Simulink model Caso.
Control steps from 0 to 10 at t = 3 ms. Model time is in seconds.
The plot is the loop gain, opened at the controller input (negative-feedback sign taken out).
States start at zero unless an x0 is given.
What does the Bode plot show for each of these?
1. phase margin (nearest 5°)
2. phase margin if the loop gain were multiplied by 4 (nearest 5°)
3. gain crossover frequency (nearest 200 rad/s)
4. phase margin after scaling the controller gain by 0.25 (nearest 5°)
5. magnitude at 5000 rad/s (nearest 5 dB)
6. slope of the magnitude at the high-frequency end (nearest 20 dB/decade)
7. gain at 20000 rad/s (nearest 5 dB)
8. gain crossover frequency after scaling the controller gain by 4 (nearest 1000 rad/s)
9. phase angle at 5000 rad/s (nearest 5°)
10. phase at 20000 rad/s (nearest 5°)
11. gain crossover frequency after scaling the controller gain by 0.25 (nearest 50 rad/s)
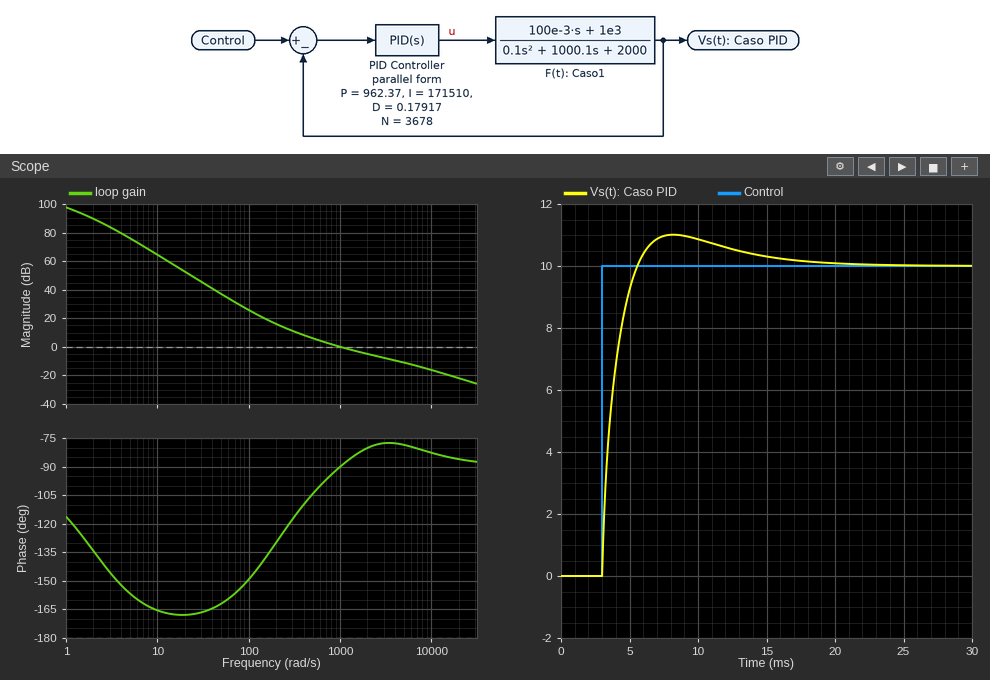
90°
100°
1000 rad/s
60°
-10 dB
-20 dB/decade
-20 dB
6000 rad/s
-80°
-85°
300 rad/s
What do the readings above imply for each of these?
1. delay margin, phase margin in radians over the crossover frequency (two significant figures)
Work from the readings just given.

0.0016 s
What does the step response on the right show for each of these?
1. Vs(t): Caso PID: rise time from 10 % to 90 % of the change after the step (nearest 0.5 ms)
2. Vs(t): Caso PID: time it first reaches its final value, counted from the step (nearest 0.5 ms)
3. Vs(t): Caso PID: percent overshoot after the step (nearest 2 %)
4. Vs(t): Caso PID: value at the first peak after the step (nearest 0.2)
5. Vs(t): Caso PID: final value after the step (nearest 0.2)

2.0 ms
2.5 ms
10 %
11.0
10.0
